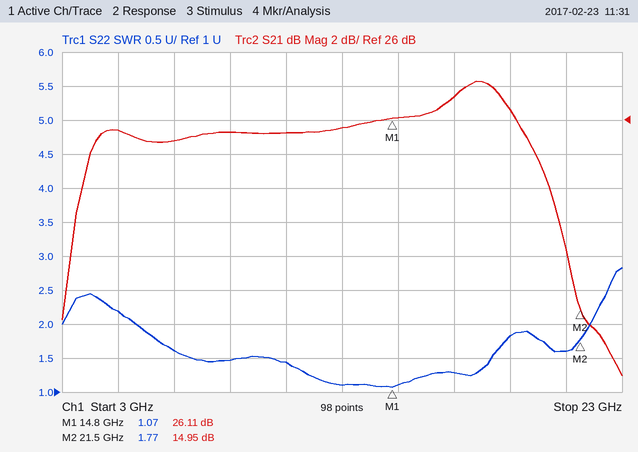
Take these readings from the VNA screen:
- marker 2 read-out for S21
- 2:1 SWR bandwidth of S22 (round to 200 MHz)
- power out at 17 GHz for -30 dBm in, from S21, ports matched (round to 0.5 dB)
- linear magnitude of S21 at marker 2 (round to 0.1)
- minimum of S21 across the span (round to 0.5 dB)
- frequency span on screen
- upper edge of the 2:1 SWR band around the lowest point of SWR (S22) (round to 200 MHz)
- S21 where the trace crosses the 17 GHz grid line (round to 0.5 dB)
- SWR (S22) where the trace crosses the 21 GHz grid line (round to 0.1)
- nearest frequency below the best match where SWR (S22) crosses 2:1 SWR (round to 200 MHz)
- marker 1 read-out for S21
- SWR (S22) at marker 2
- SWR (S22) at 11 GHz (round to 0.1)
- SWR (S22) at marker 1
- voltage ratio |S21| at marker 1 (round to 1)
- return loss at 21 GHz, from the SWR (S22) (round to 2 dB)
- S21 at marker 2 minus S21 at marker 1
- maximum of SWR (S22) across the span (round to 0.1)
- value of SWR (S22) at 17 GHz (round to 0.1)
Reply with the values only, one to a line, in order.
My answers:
14.95 dB
16.2 GHz
-2.5 dBm
5.6
11.0 dB
20 GHz
21.8 GHz
27.5 dB
1.6
5.6 GHz
26.11 dB
1.77
1.4
1.07
20
12 dB
-11.16 dB
2.8
1.3
